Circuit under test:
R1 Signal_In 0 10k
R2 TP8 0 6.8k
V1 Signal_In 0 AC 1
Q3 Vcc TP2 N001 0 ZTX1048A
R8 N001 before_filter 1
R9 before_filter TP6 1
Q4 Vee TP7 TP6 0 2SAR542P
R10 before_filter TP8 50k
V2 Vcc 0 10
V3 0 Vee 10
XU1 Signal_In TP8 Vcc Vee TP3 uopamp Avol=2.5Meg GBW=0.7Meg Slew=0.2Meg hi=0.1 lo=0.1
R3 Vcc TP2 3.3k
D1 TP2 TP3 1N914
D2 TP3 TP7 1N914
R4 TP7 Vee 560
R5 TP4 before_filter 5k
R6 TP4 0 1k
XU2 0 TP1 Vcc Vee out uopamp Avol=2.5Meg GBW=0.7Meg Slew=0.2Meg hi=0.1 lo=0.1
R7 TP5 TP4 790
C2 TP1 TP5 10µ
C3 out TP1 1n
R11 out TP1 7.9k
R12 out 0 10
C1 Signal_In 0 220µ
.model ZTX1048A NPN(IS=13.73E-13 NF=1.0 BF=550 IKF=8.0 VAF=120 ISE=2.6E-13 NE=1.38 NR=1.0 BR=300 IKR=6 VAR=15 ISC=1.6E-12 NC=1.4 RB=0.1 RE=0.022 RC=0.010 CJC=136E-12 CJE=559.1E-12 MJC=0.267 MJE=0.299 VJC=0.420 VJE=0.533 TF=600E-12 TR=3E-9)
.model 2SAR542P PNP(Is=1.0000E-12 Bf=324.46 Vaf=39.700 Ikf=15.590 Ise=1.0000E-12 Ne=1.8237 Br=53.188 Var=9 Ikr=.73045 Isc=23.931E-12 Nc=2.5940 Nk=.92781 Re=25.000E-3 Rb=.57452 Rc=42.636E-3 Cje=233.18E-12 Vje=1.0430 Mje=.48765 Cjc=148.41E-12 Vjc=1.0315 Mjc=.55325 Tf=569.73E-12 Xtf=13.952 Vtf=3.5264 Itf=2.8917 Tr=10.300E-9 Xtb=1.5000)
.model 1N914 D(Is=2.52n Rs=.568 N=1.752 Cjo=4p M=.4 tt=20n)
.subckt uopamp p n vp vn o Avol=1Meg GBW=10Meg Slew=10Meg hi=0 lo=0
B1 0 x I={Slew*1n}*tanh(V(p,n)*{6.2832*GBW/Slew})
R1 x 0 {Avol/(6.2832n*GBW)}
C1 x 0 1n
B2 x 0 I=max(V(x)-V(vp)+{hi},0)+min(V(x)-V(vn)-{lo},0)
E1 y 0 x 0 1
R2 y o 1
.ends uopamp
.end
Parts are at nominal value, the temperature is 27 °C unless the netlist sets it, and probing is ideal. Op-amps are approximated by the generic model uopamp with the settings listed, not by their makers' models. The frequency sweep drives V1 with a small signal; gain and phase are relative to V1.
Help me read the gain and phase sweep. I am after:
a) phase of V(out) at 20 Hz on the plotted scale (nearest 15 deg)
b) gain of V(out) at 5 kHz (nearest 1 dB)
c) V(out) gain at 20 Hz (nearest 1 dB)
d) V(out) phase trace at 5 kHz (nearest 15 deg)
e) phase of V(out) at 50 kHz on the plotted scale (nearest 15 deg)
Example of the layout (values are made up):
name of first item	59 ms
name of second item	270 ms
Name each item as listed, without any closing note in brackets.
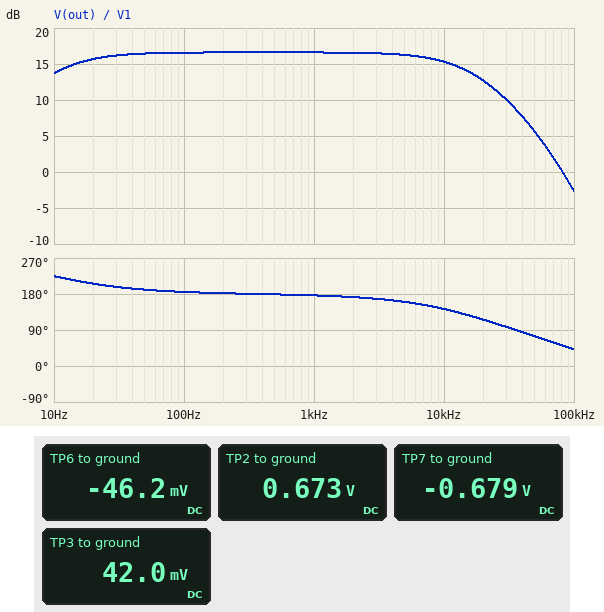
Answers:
phase of V(out) at 20 Hz on the plotted scale	210 deg
gain of V(out) at 5 kHz	16 dB
V(out) gain at 20 Hz	16 dB
V(out) phase trace at 5 kHz	165 deg
phase of V(out) at 50 kHz on the plotted scale	75 deg
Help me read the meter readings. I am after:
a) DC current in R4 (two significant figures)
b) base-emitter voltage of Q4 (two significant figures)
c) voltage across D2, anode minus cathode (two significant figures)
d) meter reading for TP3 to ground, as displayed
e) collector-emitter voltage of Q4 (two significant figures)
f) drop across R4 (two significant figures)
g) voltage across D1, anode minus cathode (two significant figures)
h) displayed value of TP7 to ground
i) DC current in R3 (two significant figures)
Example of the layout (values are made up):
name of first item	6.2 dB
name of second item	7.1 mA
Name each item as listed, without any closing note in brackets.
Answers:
DC current in R4	17 mA
base-emitter voltage of Q4	-630 mV
voltage across D2, anode minus cathode	720 mV
meter reading for TP3 to ground, as displayed	42.0 mV
collector-emitter voltage of Q4	-10 V
drop across R4	9.3 V
voltage across D1, anode minus cathode	630 mV
displayed value of TP7 to ground	-0.679 V
DC current in R3	2.8 mA
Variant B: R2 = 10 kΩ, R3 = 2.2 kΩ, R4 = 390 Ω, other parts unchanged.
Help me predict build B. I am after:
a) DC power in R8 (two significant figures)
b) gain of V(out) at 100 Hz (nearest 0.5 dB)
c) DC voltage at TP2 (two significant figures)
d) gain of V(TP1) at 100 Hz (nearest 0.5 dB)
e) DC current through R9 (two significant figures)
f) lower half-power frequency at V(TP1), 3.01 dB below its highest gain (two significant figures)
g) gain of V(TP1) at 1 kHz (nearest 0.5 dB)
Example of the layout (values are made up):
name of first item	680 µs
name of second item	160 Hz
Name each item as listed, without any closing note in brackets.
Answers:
DC power in R8	3.5 mW
gain of V(out) at 100 Hz	13.5 dB
DC voltage at TP2	690 mV
gain of V(TP1) at 100 Hz	-62.5 dB
DC current through R9	59 mA
lower half-power frequency at V(TP1), 3.01 dB below its highest gain	14 kHz
gain of V(TP1) at 1 kHz	-42.5 dB
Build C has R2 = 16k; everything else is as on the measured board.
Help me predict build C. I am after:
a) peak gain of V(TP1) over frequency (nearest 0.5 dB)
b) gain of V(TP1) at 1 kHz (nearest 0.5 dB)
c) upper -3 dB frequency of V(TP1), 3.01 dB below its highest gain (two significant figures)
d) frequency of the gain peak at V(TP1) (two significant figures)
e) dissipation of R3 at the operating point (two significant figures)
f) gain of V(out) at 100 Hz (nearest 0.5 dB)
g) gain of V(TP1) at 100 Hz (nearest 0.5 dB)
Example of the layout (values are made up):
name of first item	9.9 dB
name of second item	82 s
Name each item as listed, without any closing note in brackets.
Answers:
peak gain of V(TP1) over frequency	-21.5 dB
gain of V(TP1) at 1 kHz	-45.5 dB
upper -3 dB frequency of V(TP1), 3.01 dB below its highest gain	190 kHz
frequency of the gain peak at V(TP1)	53 kHz
dissipation of R3 at the operating point	26 mW
gain of V(out) at 100 Hz	10.5 dB
gain of V(TP1) at 100 Hz	-65.5 dB
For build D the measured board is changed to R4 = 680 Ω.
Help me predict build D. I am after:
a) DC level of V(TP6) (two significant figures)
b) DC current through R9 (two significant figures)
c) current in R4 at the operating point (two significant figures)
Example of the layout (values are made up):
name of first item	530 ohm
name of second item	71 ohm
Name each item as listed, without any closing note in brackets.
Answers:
DC level of V(TP6)	-43 mV
DC current through R9	43 mA
current in R4 at the operating point	14 mA
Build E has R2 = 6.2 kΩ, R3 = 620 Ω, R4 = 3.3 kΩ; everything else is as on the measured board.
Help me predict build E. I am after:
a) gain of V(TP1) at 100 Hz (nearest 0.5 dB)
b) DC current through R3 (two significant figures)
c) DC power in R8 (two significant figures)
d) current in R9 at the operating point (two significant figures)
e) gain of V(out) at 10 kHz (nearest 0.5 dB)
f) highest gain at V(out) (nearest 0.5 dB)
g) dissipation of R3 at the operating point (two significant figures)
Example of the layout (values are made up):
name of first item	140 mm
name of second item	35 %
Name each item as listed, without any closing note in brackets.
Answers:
gain of V(TP1) at 100 Hz	-59.0 dB
DC current through R3	15 mA
DC power in R8	2.0 mW
current in R9 at the operating point	44 mA
gain of V(out) at 10 kHz	16.0 dB
highest gain at V(out)	17.5 dB
dissipation of R3 at the operating point	140 mW
